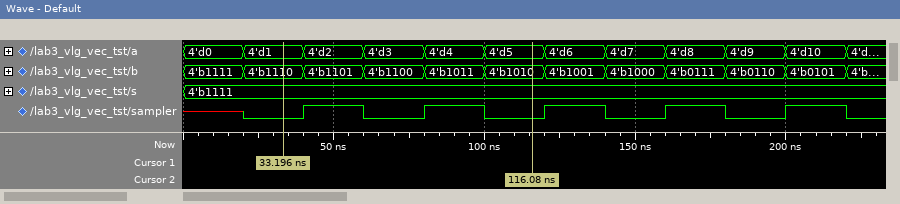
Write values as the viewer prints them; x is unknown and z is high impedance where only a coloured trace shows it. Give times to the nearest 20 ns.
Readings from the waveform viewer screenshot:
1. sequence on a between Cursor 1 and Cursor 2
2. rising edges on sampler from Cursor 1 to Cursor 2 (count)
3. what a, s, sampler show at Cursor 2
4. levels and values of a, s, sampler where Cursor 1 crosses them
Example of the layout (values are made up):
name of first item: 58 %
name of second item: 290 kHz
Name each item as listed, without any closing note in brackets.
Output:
sequence on a between Cursor 1 and Cursor 2: 4'd1, 4'd2, 4'd3, 4'd4, 4'd5
rising edges on sampler from Cursor 1 to Cursor 2: 2
what a, s, sampler show at Cursor 2: a=4'd5, s=4'b1111, sampler=0
levels and values of a, s, sampler where Cursor 1 crosses them: a=4'd1, s=4'b1111, sampler=0
